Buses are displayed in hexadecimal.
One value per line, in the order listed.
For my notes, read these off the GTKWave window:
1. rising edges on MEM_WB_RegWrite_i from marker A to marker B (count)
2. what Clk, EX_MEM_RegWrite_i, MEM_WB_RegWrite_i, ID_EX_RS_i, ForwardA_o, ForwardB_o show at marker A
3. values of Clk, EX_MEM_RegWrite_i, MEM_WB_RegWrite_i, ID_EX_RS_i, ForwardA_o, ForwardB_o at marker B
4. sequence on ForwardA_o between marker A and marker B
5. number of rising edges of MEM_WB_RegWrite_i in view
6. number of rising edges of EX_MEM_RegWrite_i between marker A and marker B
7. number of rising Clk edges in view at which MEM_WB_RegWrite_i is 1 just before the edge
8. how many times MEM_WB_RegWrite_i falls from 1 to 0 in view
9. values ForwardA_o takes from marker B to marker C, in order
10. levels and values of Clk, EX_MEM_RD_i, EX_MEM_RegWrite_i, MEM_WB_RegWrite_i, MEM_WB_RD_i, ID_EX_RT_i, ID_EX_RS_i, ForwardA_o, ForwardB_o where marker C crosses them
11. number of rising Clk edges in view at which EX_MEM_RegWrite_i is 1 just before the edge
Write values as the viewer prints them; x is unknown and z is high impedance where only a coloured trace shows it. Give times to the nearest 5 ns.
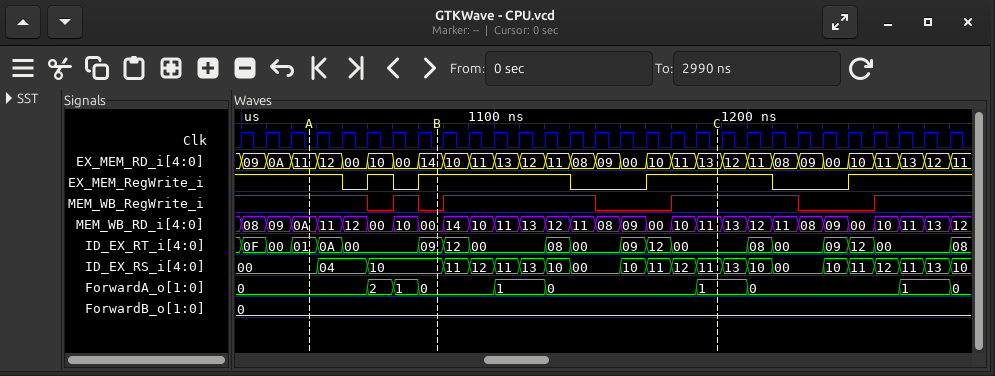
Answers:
1
Clk=0, EX_MEM_RegWrite_i=1, MEM_WB_RegWrite_i=1, ID_EX_RS_i=00, ForwardA_o=0, ForwardB_o=0
Clk=0, EX_MEM_RegWrite_i=1, MEM_WB_RegWrite_i=0, ID_EX_RS_i=10, ForwardA_o=0, ForwardB_o=0
0, 2, 1, 0
4
2
21
4
0, 1, 0, 1
Clk=0, EX_MEM_RD_i=13, EX_MEM_RegWrite_i=1, MEM_WB_RegWrite_i=1, MEM_WB_RD_i=11, ID_EX_RT_i=00, ID_EX_RS_i=11, ForwardA_o=1, ForwardB_o=0
21
